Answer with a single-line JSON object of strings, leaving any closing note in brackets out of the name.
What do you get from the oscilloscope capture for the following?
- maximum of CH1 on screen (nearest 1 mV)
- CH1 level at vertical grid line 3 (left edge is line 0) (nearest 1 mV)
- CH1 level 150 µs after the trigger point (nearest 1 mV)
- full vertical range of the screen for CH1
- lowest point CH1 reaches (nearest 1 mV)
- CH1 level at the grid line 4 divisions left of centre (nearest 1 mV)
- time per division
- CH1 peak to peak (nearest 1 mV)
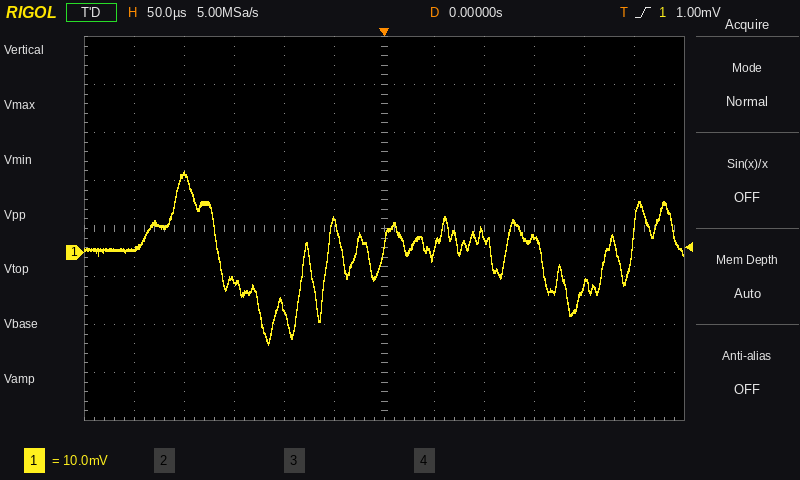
{"maximum of CH1 on screen": "17 mV", "CH1 level at vertical grid line 3 (left edge is line 0)": "-6 mV", "CH1 level 150 µs after the trigger point": "3 mV", "full vertical range of the screen for CH1": "80 mV", "lowest point CH1 reaches": "-19 mV", "CH1 level at the grid line 4 divisions left of centre": "16 mV", "time per division": "50 µs", "CH1 peak to peak": "36 mV"}
